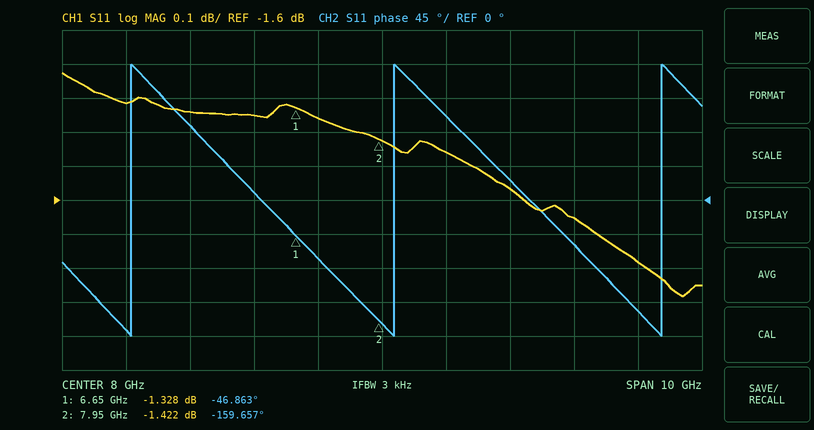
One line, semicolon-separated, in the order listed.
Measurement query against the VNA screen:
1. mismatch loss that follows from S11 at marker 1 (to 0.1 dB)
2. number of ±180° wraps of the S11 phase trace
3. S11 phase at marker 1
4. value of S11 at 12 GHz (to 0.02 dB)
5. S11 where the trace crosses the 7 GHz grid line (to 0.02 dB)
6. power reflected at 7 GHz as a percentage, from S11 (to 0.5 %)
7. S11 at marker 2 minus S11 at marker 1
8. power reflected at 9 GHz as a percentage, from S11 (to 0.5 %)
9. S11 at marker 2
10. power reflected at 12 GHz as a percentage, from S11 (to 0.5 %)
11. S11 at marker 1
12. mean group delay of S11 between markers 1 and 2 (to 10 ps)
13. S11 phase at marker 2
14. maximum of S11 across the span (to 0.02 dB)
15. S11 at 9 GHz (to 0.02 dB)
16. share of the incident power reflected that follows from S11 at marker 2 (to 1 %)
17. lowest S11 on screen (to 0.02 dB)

5.8 dB; 3; -46.863°; -1.78 dB; -1.36 dB; 73.0 %; -0.094 dB; 71.5 %; -1.422 dB; 66.5 %; -1.328 dB; 240 ps; -159.657°; -1.22 dB; -1.46 dB; 72 %; -1.88 dB
